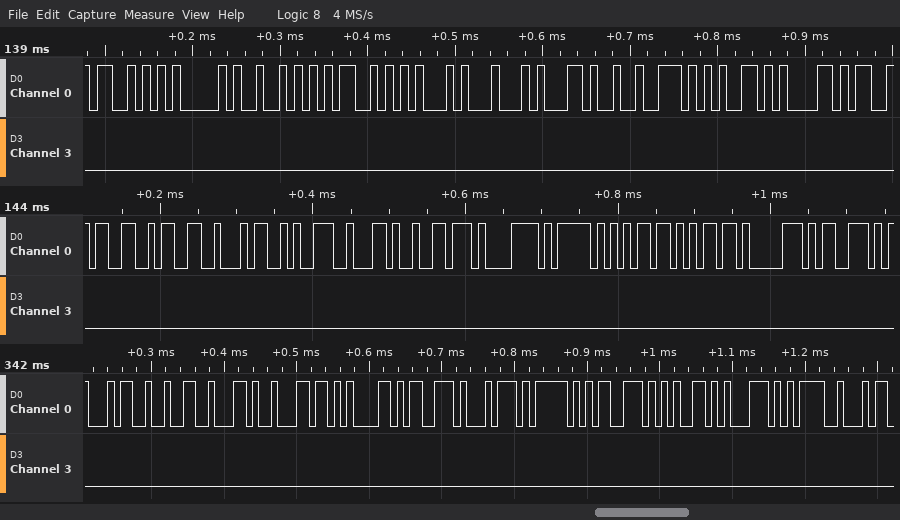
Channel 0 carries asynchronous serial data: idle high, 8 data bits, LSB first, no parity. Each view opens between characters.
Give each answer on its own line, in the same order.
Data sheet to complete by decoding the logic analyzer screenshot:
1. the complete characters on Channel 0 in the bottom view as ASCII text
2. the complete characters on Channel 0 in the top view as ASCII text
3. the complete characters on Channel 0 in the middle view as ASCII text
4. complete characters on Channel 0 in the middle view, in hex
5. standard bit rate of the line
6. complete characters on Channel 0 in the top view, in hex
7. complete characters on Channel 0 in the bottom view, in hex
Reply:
"42,last_seq="
"SARMED,rea"
"3349,vx_mmps"
33, 33, 34, 39, 2C, 76, 78, 5F, 6D, 6D, 70, 73
115200 baud
53, 41, 52, 4D, 45, 44, 2C, 72, 65, 61
34, 32, 2C, 6C, 61, 73, 74, 5F, 73, 65, 71, 3D
